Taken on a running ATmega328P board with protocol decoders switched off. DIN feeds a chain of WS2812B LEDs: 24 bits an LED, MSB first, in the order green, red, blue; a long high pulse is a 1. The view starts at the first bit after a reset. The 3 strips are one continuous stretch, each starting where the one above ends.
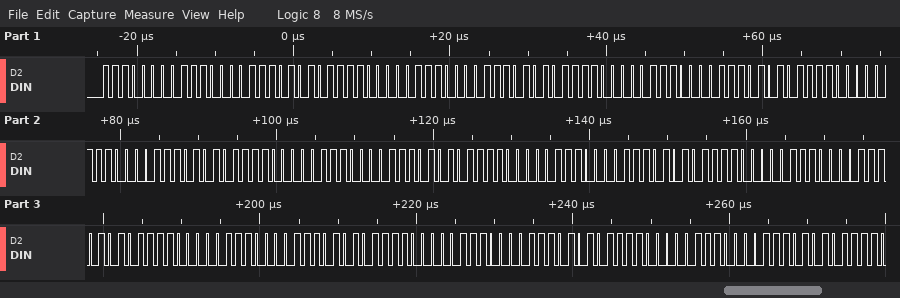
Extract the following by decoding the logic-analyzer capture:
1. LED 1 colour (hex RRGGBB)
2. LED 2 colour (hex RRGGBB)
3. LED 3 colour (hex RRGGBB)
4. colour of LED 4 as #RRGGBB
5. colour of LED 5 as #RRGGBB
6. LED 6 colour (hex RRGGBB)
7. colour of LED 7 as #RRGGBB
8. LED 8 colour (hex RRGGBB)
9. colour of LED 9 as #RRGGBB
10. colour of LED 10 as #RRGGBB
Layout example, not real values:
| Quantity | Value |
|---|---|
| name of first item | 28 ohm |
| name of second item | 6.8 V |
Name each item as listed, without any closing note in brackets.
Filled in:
| Quantity | Value |
|---|---|
| LED 1 colour | #E1E0D5 |
| LED 2 colour | #E1E0D5 |
| LED 3 colour | #E1E0D5 |
| colour of LED 4 as #RRGGBB | #E1E0D5 |
| colour of LED 5 as #RRGGBB | #E1E0D5 |
| LED 6 colour | #E1E0D5 |
| colour of LED 7 as #RRGGBB | #E1E0D5 |
| LED 8 colour | #E1E0D5 |
| colour of LED 9 as #RRGGBB | #E1E0D5 |
| colour of LED 10 as #RRGGBB | #E1E0D5 |
